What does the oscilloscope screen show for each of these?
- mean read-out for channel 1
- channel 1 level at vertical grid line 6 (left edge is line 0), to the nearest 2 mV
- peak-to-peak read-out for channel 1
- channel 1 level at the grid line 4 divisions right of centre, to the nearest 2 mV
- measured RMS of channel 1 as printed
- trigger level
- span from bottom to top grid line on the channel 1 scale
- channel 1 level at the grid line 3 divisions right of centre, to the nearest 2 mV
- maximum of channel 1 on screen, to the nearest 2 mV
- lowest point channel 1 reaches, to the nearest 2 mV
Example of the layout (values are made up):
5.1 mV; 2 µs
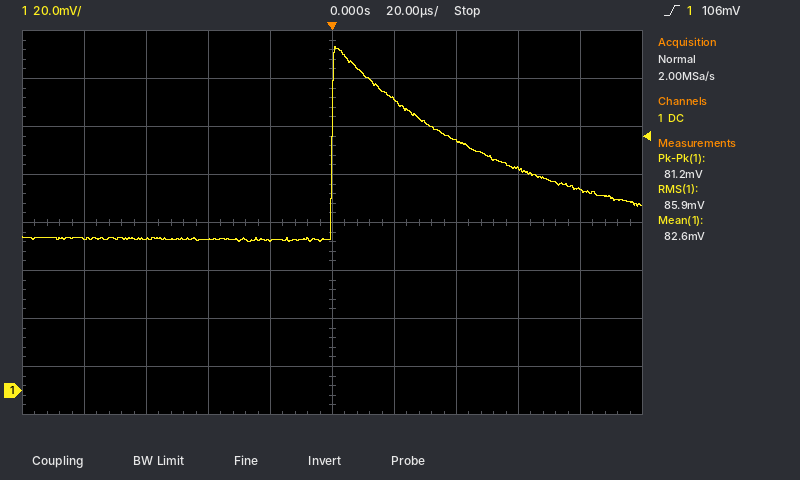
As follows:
82.6 mV; 122 mV; 81.2 mV; 84 mV; 85.9 mV; 106 mV; 160 mV; 92 mV; 144 mV; 62 mV
